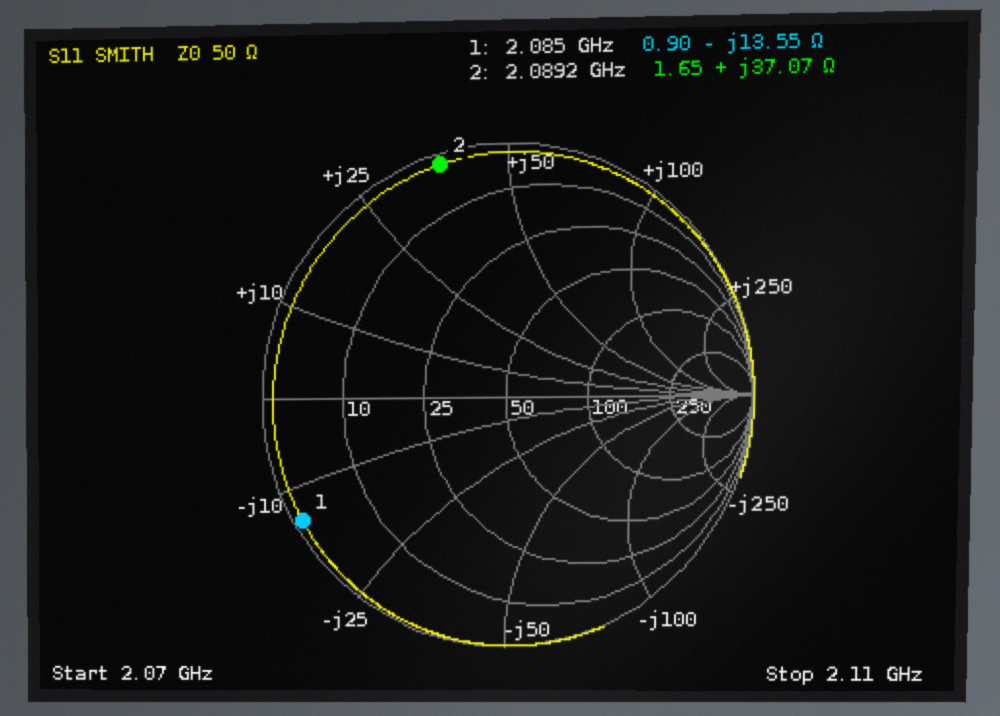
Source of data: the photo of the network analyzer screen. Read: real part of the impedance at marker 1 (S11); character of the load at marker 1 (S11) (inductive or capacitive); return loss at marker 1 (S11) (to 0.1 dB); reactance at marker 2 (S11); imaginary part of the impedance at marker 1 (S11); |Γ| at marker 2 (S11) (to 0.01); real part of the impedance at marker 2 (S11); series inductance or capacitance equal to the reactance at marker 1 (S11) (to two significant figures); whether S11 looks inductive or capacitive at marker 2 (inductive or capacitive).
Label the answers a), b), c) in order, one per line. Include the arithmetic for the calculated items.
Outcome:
a) 0.90 Ω
b) capacitive
c) 0.3 dB
d) +37.07 Ω
e) -13.55 Ω
f) 0.96
g) 1.65 Ω
h) C = 1/(2π × 2.085 GHz × 13.55 Ω) ≈ 5.6 pF
i) inductive
